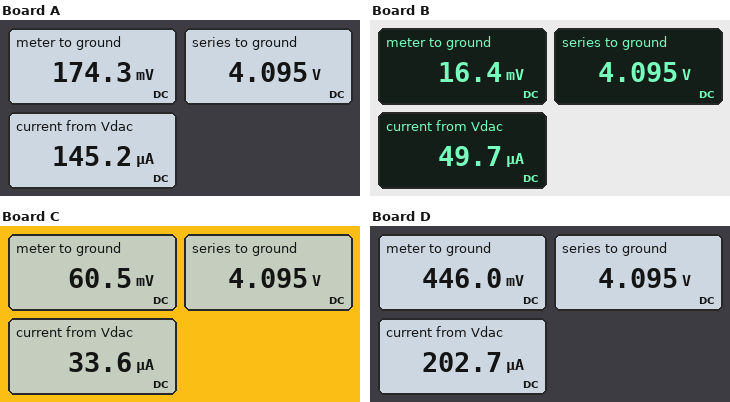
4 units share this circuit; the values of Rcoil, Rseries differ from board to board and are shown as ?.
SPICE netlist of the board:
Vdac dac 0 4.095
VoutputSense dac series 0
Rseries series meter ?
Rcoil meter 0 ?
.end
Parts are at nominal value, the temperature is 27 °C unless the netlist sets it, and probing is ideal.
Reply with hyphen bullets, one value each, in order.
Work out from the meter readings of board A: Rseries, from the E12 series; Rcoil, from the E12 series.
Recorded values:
- 27 kΩ
- 1.2 kΩ
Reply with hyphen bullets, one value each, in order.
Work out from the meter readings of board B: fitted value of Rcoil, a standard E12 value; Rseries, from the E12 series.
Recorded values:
- 330 Ω
- 82 kΩ
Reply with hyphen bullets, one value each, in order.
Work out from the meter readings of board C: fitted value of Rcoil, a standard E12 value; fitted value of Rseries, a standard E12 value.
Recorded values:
- 1.8 kΩ
- 120 kΩ
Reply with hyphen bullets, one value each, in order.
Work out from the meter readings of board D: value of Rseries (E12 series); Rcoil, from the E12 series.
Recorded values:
- 18 kΩ
- 2.2 kΩ
